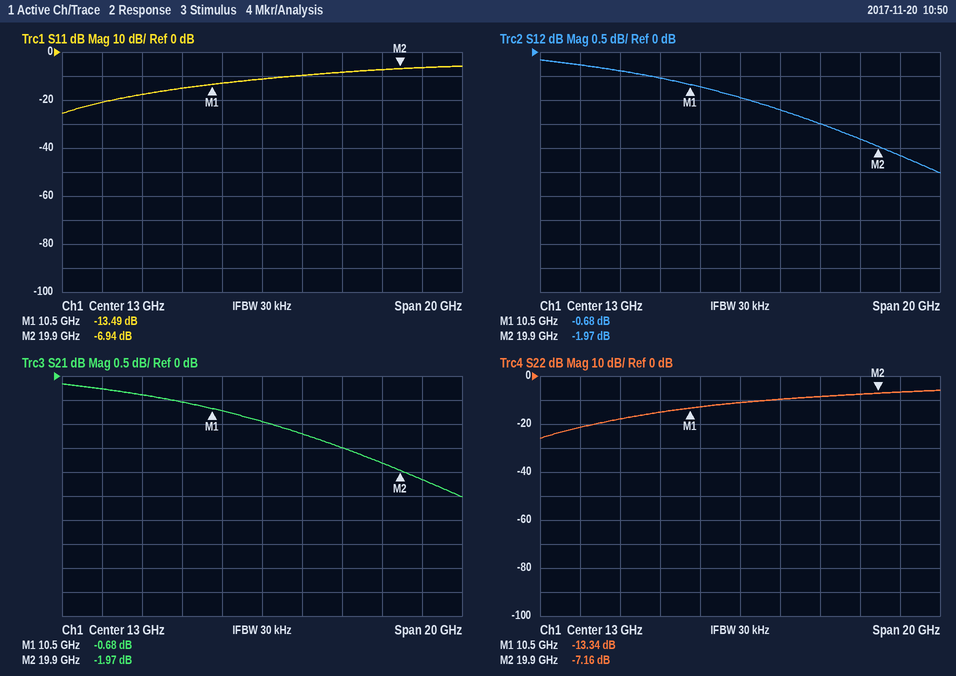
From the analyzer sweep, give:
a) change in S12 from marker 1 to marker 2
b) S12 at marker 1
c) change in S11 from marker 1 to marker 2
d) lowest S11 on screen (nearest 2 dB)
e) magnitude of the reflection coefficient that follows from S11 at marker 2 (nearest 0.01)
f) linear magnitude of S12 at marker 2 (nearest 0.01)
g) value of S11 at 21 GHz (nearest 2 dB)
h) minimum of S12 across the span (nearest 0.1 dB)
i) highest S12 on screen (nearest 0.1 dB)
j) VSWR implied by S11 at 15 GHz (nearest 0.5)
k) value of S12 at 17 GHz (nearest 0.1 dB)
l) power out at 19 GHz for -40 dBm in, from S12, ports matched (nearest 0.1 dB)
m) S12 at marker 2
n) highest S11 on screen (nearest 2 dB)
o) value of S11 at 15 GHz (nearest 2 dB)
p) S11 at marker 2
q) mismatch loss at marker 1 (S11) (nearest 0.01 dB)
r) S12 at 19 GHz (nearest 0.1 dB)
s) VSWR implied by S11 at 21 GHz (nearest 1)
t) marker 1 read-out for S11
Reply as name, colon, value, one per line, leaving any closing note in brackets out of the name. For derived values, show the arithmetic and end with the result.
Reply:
change in S12 from marker 1 to marker 2: -1.97 − (-0.68) = -1.29 dB
S12 at marker 1: -0.68 dB
change in S11 from marker 1 to marker 2: -6.94 − (-13.49) = 6.55 dB
lowest S11 on screen: -26 dB
magnitude of the reflection coefficient that follows from S11 at marker 2: 10^(-6.94/20) ≈ 0.45
linear magnitude of S12 at marker 2: 10^(-1.97/20) ≈ 0.80
value of S11 at 21 GHz: -6 dB
minimum of S12 across the span: -2.5 dB
highest S12 on screen: -0.2 dB
VSWR implied by S11 at 15 GHz: |Γ| = 10^(-10/20) = 0.3162; VSWR = (1 + 0.3162)/(1 − 0.3162) ≈ 1.92, so 2.0 to the nearest 0.5
value of S12 at 17 GHz: -1.5 dB
power out at 19 GHz for -40 dBm in, from S12, ports matched: -40 dBm + (-1.8 dB) = -41.8 dBm
S12 at marker 2: -1.97 dB
highest S11 on screen: -6 dB
value of S11 at 15 GHz: -10 dB
S11 at marker 2: -6.94 dB
mismatch loss at marker 1 (S11): −10 log10(1 − 10^(-13.49/10)) ≈ 0.20 dB
S12 at 19 GHz: -1.8 dB
VSWR implied by S11 at 21 GHz: |Γ| = 10^(-6/20) = 0.5012; VSWR = (1 + 0.5012)/(1 − 0.5012) ≈ 3
marker 1 read-out for S11: -13.49 dB
